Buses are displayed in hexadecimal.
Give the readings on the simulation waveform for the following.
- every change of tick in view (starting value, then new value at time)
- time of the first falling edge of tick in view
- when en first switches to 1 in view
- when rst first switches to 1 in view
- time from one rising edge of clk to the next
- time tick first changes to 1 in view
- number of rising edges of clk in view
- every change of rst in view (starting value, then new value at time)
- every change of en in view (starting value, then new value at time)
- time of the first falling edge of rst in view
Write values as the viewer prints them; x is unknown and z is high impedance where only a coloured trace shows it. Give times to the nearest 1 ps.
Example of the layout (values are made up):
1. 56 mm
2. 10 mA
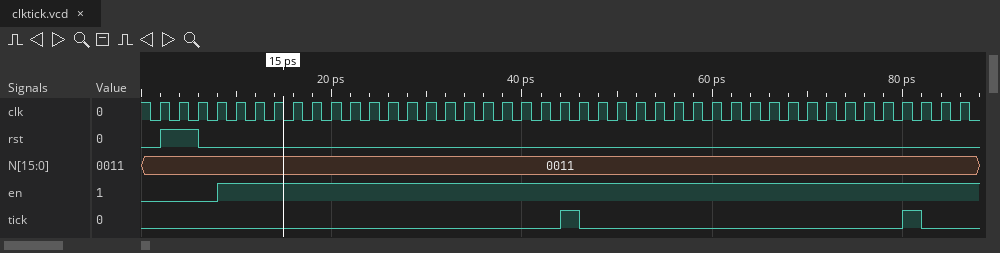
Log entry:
1. 0, 1 at 44 ps, 0 at 46 ps, 1 at 80 ps, 0 at 82 ps
2. 46 ps
3. 8 ps
4. 2 ps
5. 2 ps
6. 44 ps
7. 43
8. 0, 1 at 2 ps, 0 at 6 ps
9. 0, 1 at 8 ps
10. 6 ps
